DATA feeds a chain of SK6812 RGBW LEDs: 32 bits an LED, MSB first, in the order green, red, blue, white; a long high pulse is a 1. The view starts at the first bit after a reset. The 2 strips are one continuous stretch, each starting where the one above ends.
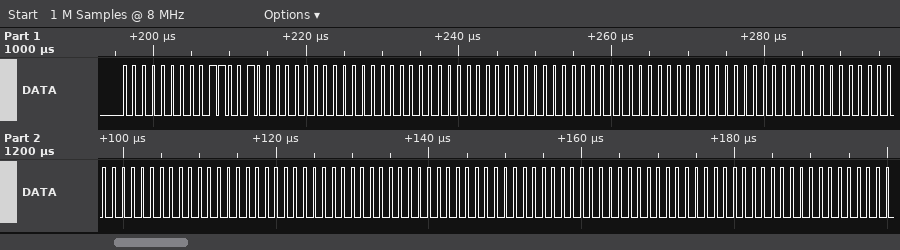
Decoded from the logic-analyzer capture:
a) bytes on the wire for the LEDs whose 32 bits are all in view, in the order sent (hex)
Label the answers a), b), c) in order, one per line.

a) 00 64 00 00 00 00 00 00 00 00 00 00 00 00 00 00 00 00 00 00
